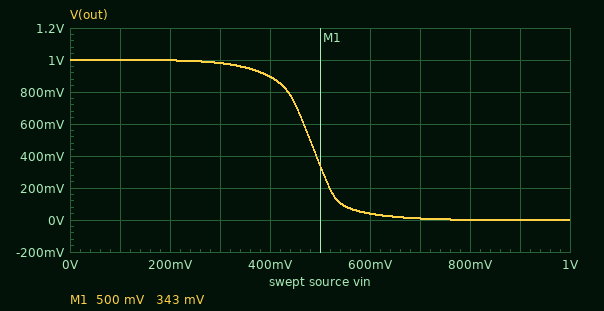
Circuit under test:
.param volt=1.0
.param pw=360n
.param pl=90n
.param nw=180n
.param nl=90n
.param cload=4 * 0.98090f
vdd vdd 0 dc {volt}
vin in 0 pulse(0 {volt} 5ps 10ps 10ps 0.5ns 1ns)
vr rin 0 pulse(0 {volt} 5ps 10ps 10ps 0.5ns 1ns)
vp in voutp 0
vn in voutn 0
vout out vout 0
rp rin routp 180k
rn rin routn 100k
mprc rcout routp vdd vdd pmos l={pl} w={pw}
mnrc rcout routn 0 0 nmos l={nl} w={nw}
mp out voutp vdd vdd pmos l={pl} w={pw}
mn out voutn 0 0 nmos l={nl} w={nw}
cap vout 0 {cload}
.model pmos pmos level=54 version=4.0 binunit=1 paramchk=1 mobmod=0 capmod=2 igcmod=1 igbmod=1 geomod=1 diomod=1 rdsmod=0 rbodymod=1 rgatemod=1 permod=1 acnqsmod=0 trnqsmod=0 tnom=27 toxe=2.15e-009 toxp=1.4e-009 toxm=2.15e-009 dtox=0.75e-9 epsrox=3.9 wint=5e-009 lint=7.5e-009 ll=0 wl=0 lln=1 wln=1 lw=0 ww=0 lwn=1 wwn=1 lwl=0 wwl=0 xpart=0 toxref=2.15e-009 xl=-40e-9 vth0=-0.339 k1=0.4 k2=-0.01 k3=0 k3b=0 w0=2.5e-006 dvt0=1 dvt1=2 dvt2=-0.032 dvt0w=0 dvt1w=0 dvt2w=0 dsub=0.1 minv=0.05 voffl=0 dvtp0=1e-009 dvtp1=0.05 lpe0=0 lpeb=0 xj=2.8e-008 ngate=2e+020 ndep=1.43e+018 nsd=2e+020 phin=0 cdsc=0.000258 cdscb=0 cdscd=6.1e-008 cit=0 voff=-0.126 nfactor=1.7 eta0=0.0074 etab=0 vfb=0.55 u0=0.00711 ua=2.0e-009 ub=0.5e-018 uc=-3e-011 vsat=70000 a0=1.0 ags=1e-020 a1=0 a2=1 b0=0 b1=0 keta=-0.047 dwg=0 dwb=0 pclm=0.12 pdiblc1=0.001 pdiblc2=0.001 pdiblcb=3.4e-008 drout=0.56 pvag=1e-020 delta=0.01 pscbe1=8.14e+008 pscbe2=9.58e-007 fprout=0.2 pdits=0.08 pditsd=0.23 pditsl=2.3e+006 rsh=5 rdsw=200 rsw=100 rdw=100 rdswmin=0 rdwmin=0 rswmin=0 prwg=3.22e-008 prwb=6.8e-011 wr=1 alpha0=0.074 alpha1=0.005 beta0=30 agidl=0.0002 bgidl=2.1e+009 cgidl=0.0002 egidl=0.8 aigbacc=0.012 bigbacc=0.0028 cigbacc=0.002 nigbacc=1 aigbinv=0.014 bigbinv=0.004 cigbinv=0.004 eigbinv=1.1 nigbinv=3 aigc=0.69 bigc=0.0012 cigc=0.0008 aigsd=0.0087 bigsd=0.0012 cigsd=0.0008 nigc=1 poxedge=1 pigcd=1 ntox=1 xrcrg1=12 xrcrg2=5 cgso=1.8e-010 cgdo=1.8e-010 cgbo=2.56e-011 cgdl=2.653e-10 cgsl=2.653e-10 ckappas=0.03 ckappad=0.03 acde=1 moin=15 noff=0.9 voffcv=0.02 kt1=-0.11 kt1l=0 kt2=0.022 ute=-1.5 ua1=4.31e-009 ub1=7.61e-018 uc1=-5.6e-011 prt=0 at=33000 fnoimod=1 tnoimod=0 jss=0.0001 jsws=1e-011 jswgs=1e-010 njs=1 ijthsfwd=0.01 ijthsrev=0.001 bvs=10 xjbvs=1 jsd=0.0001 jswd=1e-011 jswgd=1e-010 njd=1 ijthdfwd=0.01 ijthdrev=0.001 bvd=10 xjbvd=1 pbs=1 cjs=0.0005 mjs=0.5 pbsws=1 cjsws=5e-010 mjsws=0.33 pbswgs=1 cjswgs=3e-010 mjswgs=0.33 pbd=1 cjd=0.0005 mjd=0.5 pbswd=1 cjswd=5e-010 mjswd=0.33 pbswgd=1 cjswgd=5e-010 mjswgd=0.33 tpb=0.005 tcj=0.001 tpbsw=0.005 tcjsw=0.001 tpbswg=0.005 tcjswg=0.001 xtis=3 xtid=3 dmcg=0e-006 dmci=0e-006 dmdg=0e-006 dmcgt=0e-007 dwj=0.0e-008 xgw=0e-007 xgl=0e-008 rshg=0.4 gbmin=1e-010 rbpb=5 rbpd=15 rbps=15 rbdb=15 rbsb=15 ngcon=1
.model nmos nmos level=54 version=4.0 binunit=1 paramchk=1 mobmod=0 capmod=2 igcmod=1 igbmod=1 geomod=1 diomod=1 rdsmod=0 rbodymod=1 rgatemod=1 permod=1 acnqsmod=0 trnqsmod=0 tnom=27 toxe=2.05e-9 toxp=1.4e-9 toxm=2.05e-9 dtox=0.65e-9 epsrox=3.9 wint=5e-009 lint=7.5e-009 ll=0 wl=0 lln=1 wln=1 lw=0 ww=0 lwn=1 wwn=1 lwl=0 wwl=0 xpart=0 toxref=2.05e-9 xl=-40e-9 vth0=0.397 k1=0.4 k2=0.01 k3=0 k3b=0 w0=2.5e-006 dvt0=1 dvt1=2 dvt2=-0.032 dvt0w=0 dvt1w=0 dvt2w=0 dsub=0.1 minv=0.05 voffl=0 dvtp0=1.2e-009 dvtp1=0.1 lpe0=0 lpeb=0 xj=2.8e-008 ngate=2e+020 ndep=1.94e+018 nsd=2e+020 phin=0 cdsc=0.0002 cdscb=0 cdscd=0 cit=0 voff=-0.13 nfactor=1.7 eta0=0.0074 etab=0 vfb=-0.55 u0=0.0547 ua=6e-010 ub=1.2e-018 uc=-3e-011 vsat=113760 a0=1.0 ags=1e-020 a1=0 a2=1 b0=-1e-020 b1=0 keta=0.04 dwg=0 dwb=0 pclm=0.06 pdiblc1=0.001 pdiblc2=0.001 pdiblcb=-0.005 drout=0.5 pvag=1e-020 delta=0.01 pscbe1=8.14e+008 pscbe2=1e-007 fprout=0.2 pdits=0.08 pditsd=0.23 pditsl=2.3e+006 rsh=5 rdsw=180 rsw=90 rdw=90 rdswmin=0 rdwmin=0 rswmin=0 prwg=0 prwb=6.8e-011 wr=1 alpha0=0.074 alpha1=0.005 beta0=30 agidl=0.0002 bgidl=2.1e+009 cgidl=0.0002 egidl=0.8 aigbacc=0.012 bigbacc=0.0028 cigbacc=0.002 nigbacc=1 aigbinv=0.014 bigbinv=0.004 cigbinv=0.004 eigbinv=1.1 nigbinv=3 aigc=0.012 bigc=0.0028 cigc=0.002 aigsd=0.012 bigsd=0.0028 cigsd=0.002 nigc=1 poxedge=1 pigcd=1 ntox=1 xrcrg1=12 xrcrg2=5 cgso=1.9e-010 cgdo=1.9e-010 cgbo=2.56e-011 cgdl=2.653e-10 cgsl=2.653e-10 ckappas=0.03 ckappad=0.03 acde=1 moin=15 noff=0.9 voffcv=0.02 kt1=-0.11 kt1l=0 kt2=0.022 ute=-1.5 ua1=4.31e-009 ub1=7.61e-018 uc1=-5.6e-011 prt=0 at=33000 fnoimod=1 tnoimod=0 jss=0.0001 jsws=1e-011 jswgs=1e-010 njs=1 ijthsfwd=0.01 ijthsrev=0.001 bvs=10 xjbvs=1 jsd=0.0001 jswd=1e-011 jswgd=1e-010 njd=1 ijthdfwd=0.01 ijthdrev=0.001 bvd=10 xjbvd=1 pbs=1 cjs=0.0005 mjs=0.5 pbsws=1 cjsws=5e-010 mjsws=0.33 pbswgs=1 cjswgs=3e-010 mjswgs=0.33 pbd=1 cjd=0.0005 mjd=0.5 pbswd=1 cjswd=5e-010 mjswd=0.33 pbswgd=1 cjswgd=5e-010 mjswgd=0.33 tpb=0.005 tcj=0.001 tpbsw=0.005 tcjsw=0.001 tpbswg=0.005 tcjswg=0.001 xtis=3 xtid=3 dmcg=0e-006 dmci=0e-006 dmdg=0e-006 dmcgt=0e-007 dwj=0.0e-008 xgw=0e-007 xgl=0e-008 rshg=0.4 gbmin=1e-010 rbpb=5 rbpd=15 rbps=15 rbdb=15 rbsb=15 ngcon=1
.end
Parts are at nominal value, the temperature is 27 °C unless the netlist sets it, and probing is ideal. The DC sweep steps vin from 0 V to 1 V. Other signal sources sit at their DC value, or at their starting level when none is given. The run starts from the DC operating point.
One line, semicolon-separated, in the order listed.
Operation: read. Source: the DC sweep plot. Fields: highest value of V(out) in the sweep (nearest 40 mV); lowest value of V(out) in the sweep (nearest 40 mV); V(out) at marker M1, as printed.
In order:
1.00 V; 0 V; 343 mV
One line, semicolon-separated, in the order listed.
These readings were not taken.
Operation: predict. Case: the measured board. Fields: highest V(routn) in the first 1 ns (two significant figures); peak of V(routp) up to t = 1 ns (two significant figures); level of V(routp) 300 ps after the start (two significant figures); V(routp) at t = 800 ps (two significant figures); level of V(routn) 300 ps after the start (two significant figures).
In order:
1.0 V; 1.0 V; 960 mV; 100 mV; 1.0 V
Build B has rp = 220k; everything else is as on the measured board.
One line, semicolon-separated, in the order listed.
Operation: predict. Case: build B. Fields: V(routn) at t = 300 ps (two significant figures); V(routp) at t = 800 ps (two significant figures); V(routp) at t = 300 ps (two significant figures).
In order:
1.0 V; 160 mV; 910 mV
